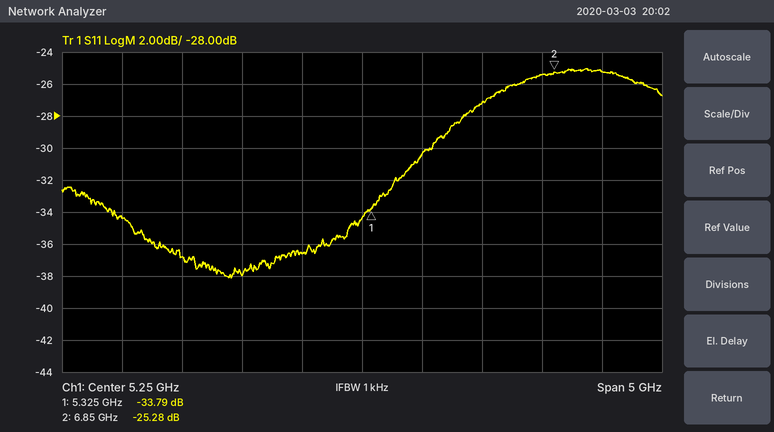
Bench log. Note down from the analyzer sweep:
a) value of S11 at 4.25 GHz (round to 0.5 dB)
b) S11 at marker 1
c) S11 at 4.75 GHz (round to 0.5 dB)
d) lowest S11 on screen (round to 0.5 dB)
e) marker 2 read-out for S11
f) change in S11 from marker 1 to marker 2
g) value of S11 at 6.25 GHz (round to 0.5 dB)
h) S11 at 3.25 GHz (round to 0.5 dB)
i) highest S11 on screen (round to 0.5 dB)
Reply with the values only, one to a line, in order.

-38.0 dB
-33.79 dB
-36.5 dB
-38.0 dB
-25.28 dB
8.51 dB
-27.0 dB
-34.5 dB
-25.0 dB
